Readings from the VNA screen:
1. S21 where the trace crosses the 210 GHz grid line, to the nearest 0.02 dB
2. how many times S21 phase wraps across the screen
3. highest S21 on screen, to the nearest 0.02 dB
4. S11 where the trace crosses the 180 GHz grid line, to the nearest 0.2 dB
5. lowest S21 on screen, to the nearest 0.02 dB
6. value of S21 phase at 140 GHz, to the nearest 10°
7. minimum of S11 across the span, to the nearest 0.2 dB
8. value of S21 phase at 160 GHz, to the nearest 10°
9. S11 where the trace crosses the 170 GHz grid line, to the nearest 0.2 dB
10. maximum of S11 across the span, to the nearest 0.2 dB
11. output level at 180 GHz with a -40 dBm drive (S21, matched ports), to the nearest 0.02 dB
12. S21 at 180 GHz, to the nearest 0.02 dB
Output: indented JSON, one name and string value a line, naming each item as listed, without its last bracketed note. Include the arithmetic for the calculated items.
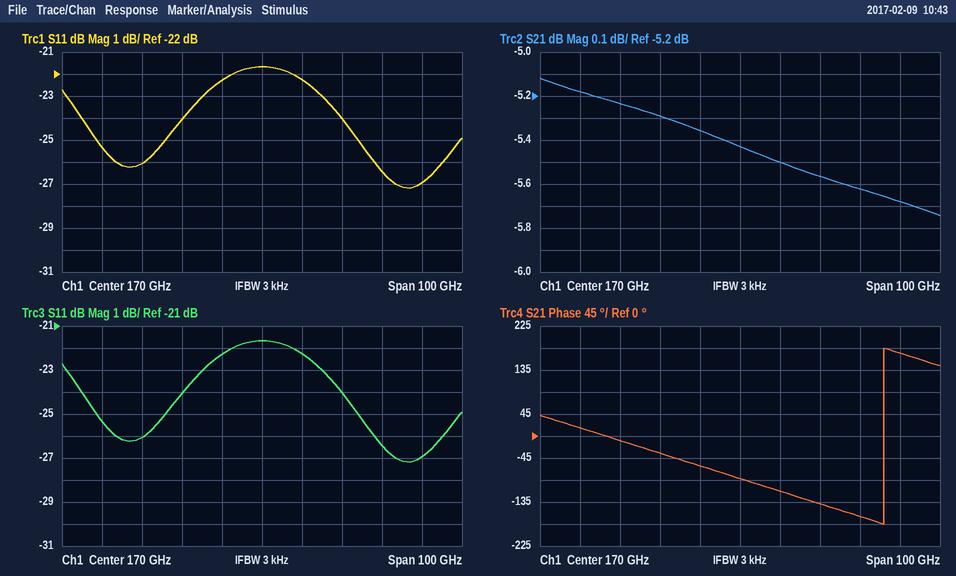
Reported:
{
  "S21 where the trace crosses the 210 GHz grid line, to the nearest 0.02 dB": "-5.68 dB",
  "how many times S21 phase wraps across the screen": "1",
  "highest S21 on screen, to the nearest 0.02 dB": "-5.12 dB",
  "S11 where the trace crosses the 180 GHz grid line, to the nearest 0.2 dB": "-22.2 dB",
  "lowest S21 on screen, to the nearest 0.02 dB": "-5.74 dB",
  "value of S21 phase at 140 GHz, to the nearest 10°": "-10°",
  "minimum of S11 across the span, to the nearest 0.2 dB": "-27.2 dB",
  "value of S21 phase at 160 GHz, to the nearest 10°": "-60°",
  "S11 where the trace crosses the 170 GHz grid line, to the nearest 0.2 dB": "-21.6 dB",
  "maximum of S11 across the span, to the nearest 0.2 dB": "-21.6 dB",
  "output level at 180 GHz with a -40 dBm drive (S21, matched ports), to the nearest 0.02 dB": "-40 dBm + (-5.50 dB) = -45.50 dBm",
  "S21 at 180 GHz, to the nearest 0.02 dB": "-5.50 dB"
}
